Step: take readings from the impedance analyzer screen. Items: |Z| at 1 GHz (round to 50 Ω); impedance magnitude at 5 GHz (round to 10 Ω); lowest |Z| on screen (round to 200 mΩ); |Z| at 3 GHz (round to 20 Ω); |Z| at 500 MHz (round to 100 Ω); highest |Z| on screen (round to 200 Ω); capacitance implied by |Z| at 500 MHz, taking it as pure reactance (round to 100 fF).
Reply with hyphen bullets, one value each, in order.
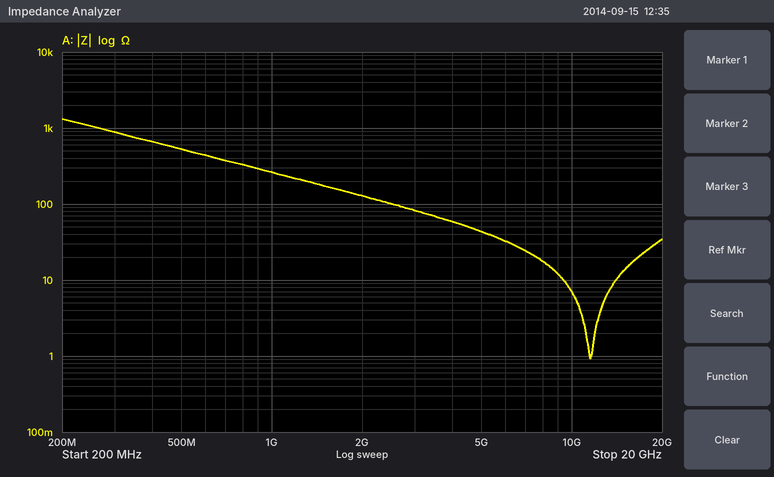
- 250 Ω
- 40 Ω
- 1.0 Ω
- 80 Ω
- 500 Ω
- 1.4 kΩ
- 600 fF
